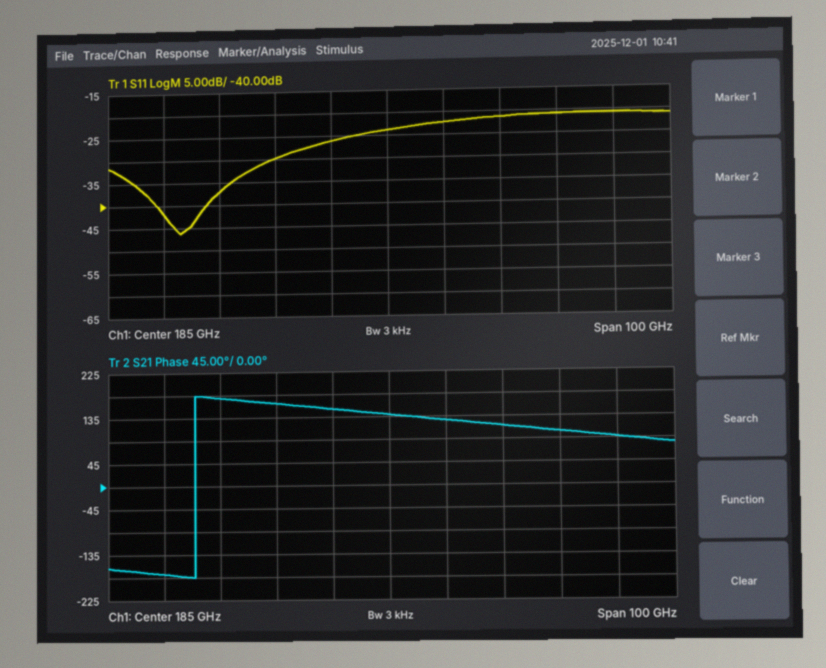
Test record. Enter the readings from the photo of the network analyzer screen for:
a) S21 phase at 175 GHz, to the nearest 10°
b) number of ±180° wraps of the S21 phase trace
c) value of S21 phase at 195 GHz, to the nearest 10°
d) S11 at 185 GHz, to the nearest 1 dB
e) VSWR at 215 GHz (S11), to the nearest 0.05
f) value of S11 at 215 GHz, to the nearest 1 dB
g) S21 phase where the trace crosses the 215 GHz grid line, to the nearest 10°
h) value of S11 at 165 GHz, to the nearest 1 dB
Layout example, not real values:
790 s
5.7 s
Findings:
150°
1
130°
-24 dB
1.20
-21 dB
100°
-30 dB
